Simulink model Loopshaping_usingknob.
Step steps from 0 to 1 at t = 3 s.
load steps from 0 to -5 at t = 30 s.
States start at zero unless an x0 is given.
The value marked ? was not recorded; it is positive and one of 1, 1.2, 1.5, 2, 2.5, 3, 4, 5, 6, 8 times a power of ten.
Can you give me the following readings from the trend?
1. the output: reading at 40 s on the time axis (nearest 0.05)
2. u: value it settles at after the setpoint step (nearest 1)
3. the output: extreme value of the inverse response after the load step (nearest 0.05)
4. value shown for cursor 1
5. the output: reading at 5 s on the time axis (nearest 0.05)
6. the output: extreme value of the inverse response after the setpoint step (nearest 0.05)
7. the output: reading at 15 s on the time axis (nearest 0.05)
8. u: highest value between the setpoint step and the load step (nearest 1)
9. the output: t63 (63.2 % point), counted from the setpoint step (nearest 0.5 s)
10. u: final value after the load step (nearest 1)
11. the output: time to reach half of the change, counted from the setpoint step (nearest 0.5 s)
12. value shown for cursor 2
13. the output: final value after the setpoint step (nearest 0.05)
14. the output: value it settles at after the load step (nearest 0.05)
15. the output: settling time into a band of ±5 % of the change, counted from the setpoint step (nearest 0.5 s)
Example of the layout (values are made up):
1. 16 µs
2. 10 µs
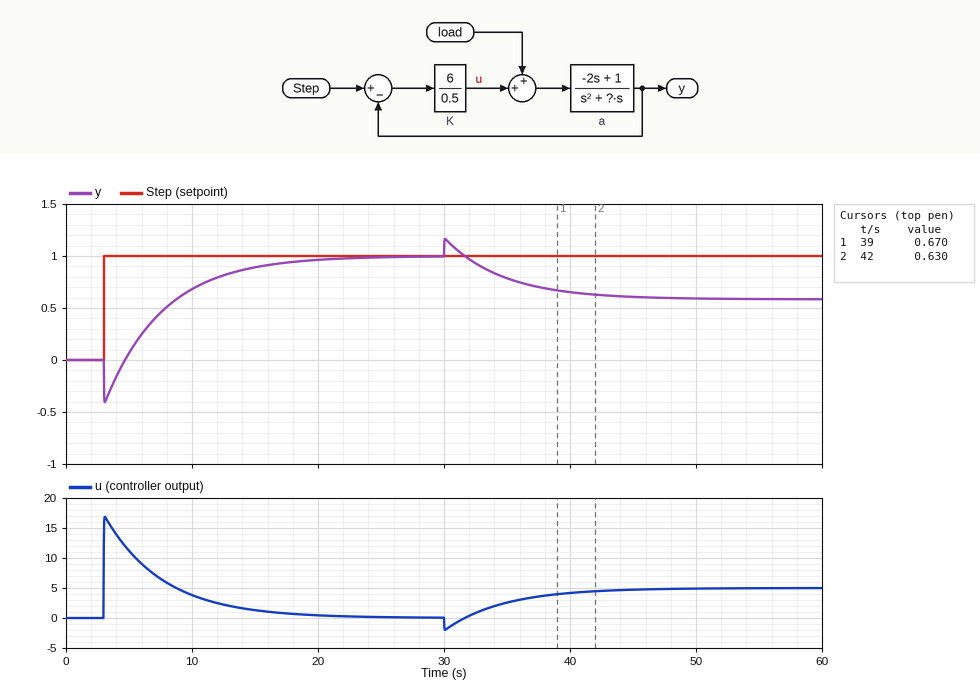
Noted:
1. 0.65
2. 0
3. 1.15
4. 0.670
5. 0.05
6. -0.40
7. 0.90
8. 17
9. 6.5 s
10. 5
11. 5.0 s
12. 0.630
13. 1.00
14. 0.60
15. 15.5 s
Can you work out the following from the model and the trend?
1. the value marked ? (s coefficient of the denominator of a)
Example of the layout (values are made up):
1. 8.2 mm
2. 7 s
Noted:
1. 80
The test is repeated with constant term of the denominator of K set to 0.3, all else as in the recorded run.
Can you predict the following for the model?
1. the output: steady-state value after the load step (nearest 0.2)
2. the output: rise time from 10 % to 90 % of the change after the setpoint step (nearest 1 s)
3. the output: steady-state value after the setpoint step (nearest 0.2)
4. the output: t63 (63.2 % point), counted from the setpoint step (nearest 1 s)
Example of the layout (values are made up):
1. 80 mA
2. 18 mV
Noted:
1. 0.8
2. 4 s
3. 1.0
4. 3 s
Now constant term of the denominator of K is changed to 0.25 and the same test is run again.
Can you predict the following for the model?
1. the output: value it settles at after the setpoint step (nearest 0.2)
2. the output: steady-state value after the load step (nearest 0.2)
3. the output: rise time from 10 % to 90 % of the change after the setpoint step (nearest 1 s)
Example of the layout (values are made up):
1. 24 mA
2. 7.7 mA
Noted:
1. 1.0
2. 0.8
3. 3 s
